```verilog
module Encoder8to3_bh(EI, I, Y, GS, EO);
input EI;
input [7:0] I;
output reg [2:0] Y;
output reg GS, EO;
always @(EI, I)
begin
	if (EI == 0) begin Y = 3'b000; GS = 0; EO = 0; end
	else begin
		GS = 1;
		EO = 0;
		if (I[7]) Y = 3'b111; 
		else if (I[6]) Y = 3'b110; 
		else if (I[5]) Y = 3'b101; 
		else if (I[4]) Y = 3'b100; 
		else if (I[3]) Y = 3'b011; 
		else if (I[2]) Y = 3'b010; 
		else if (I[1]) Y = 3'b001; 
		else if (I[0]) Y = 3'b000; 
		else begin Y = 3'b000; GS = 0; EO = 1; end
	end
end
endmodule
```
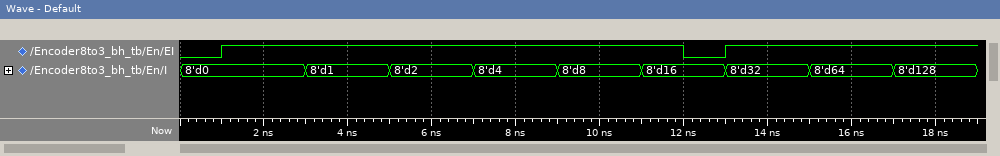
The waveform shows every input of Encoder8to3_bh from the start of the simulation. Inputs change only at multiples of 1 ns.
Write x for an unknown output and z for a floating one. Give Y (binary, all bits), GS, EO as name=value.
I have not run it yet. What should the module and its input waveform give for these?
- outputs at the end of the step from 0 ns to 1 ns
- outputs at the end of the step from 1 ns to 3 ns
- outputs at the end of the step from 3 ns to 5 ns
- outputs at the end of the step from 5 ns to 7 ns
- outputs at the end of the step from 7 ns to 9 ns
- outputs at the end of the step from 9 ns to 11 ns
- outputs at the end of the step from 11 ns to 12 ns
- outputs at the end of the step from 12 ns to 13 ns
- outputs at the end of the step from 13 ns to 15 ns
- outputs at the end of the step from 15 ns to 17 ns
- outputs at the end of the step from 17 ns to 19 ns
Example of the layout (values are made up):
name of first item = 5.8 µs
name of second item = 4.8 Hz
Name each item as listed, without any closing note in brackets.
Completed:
outputs at the end of the step from 0 ns to 1 ns = Y=000, GS=0, EO=0
outputs at the end of the step from 1 ns to 3 ns = Y=000, GS=0, EO=1
outputs at the end of the step from 3 ns to 5 ns = Y=000, GS=1, EO=0
outputs at the end of the step from 5 ns to 7 ns = Y=001, GS=1, EO=0
outputs at the end of the step from 7 ns to 9 ns = Y=010, GS=1, EO=0
outputs at the end of the step from 9 ns to 11 ns = Y=011, GS=1, EO=0
outputs at the end of the step from 11 ns to 12 ns = Y=100, GS=1, EO=0
outputs at the end of the step from 12 ns to 13 ns = Y=000, GS=0, EO=0
outputs at the end of the step from 13 ns to 15 ns = Y=101, GS=1, EO=0
outputs at the end of the step from 15 ns to 17 ns = Y=110, GS=1, EO=0
outputs at the end of the step from 17 ns to 19 ns = Y=111, GS=1, EO=0
